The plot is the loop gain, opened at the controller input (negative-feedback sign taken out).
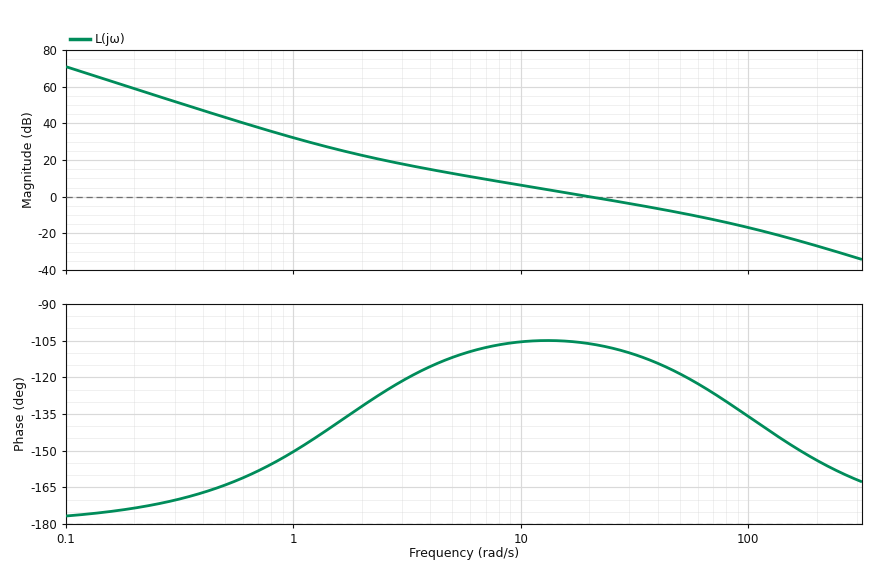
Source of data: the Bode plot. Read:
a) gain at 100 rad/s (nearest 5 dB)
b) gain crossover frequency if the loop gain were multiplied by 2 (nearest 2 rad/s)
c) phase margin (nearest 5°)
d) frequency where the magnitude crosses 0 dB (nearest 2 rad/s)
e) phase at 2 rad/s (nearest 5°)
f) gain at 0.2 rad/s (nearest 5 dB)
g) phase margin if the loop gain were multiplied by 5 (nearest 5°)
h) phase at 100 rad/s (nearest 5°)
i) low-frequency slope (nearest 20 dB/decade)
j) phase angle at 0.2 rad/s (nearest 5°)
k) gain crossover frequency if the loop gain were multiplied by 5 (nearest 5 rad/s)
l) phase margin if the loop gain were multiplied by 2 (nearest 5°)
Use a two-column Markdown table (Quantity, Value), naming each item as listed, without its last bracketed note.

| Quantity | Value |
|---|---|
| gain at 100 rad/s | -15 dB |
| gain crossover frequency if the loop gain were multiplied by 2 | 38 rad/s |
| phase margin | 75° |
| frequency where the magnitude crosses 0 dB | 20 rad/s |
| phase at 2 rad/s | -130° |
| gain at 0.2 rad/s | 60 dB |
| phase margin if the loop gain were multiplied by 5 | 50° |
| phase at 100 rad/s | -135° |
| low-frequency slope | -40 dB/decade |
| phase angle at 0.2 rad/s | -175° |
| gain crossover frequency if the loop gain were multiplied by 5 | 80 rad/s |
| phase margin if the loop gain were multiplied by 2 | 65° |
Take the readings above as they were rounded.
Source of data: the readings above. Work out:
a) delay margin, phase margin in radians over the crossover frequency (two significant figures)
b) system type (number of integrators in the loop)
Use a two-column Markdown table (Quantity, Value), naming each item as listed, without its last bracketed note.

| Quantity | Value |
|---|---|
| delay margin, phase margin in radians over the crossover frequency | 0.065 s |
| system type | 2 |
